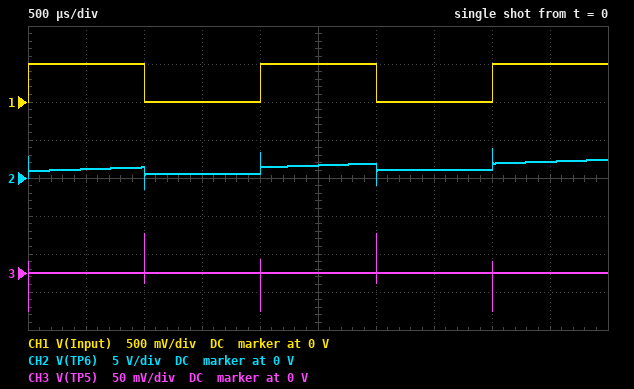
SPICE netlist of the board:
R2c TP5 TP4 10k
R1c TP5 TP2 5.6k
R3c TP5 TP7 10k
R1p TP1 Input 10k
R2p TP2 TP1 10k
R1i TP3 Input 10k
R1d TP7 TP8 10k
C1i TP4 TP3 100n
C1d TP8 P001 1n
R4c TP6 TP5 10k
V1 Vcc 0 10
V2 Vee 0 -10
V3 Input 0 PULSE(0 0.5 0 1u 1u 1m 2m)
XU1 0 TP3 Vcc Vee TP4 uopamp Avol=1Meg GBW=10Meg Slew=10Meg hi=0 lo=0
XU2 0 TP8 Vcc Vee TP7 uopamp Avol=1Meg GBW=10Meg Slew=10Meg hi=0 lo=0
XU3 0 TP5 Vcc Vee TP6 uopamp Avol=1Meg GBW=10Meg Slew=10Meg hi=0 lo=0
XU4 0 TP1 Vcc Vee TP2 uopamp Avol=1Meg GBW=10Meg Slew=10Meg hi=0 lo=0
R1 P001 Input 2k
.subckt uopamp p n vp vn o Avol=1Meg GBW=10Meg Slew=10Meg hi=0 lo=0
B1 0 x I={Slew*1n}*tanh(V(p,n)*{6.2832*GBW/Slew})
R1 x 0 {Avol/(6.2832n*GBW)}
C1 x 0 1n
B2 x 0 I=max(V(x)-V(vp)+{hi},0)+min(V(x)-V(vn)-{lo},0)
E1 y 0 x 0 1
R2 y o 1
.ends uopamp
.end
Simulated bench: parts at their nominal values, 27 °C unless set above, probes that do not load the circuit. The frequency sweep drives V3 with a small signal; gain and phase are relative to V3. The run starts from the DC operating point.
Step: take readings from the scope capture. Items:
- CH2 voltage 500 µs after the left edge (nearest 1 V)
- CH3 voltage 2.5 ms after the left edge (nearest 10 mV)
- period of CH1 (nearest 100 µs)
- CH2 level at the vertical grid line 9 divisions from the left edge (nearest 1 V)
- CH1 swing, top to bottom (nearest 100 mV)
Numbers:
1 V
0 V
2.0 ms
2 V
500 mV
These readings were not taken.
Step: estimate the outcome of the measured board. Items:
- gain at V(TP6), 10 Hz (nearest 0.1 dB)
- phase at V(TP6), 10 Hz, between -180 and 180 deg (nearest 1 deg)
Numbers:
24.1 dB
-84 deg
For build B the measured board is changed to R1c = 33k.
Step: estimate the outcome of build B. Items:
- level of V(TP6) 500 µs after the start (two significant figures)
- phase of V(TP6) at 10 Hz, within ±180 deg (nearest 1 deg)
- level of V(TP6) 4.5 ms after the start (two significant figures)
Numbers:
400 mV
-89 deg
1.4 V
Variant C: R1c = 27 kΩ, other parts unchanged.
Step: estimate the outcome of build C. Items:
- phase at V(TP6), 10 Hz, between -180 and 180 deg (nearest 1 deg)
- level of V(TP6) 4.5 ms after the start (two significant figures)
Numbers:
-89 deg
1.4 V
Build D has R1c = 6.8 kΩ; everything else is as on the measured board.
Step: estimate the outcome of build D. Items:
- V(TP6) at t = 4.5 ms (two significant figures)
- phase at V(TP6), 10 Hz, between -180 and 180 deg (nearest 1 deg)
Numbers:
2.0 V
-85 deg
